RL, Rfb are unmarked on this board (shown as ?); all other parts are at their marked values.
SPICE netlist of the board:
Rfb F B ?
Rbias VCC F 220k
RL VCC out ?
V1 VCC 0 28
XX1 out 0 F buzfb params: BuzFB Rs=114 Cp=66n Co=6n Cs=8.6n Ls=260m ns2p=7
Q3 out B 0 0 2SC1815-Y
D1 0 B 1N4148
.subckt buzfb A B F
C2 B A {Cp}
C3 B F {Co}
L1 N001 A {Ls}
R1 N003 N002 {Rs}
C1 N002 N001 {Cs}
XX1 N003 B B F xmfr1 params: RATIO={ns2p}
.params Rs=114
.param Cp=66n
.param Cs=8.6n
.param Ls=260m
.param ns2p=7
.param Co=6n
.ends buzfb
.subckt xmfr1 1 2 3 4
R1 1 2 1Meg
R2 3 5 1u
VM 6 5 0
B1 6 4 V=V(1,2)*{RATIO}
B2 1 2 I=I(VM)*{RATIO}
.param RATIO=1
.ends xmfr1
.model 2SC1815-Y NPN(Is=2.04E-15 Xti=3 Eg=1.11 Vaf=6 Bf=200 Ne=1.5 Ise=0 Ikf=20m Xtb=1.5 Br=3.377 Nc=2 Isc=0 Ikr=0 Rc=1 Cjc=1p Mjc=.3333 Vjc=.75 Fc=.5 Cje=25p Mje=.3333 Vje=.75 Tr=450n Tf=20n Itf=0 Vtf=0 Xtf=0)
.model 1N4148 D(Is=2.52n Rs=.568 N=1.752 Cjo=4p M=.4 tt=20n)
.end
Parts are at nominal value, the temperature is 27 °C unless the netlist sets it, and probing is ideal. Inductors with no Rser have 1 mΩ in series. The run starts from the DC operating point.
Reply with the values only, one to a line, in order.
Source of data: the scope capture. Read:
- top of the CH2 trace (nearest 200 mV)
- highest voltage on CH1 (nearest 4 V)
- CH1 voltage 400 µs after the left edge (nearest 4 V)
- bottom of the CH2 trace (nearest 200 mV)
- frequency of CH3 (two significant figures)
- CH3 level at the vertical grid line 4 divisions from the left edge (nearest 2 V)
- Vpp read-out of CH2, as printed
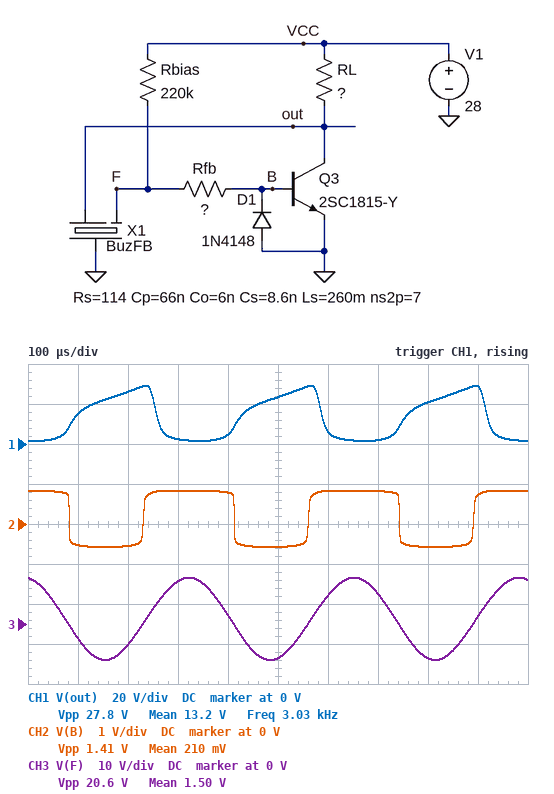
800 mV
28 V
4 V
-600 mV
3.0 kHz
2 V
1.41 V
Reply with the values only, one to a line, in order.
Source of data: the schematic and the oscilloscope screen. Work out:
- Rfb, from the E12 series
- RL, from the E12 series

10 kΩ
470 Ω
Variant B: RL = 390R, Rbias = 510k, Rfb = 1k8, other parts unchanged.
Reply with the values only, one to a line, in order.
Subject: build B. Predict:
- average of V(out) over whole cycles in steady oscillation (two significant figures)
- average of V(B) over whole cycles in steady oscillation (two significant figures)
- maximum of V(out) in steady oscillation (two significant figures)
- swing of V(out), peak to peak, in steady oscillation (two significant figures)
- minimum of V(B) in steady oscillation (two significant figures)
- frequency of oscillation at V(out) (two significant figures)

8.4 V
120 mV
26 V
25 V
-670 mV
3.3 kHz
